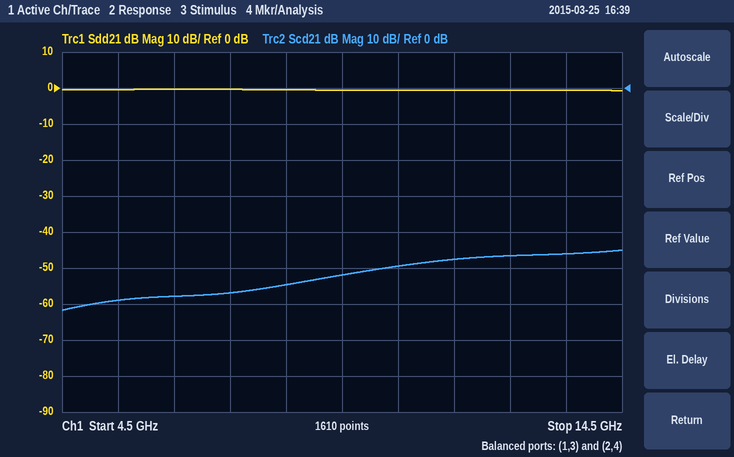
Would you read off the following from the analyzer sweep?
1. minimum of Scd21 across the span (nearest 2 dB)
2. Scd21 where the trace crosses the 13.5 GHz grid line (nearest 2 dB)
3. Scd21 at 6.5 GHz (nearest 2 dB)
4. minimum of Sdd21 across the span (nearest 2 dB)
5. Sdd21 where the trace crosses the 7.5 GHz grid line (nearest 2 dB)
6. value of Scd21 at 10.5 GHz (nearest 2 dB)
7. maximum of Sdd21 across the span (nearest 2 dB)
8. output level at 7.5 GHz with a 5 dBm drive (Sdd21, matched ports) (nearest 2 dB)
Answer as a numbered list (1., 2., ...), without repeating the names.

1. -62 dB
2. -46 dB
3. -58 dB
4. 0 dB
5. 0 dB
6. -50 dB
7. 0 dB
8. 4 dBm
